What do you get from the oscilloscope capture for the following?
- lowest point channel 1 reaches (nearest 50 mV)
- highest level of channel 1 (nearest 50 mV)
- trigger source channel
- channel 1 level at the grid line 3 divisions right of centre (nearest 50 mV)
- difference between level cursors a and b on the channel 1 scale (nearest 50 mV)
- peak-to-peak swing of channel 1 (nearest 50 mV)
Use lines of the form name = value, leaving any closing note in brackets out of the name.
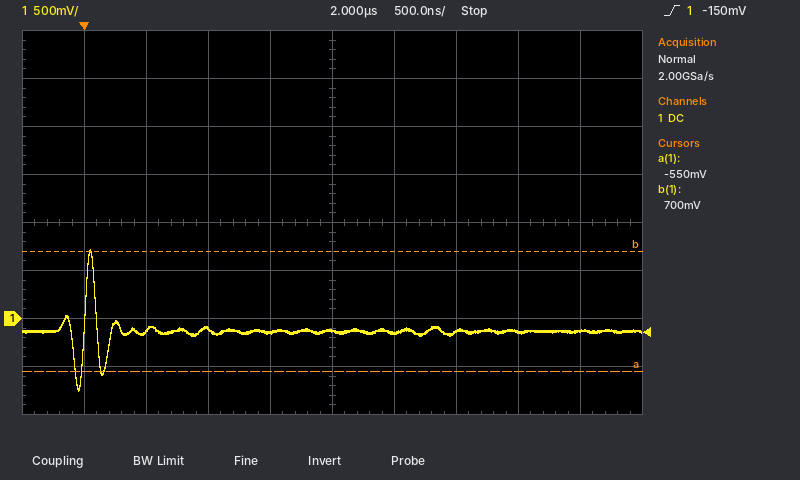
lowest point channel 1 reaches = -750 mV
highest level of channel 1 = 700 mV
trigger source channel = channel 1
channel 1 level at the grid line 3 divisions right of centre = -150 mV
difference between level cursors a and b on the channel 1 scale = 1.25 V
peak-to-peak swing of channel 1 = 1.45 V
